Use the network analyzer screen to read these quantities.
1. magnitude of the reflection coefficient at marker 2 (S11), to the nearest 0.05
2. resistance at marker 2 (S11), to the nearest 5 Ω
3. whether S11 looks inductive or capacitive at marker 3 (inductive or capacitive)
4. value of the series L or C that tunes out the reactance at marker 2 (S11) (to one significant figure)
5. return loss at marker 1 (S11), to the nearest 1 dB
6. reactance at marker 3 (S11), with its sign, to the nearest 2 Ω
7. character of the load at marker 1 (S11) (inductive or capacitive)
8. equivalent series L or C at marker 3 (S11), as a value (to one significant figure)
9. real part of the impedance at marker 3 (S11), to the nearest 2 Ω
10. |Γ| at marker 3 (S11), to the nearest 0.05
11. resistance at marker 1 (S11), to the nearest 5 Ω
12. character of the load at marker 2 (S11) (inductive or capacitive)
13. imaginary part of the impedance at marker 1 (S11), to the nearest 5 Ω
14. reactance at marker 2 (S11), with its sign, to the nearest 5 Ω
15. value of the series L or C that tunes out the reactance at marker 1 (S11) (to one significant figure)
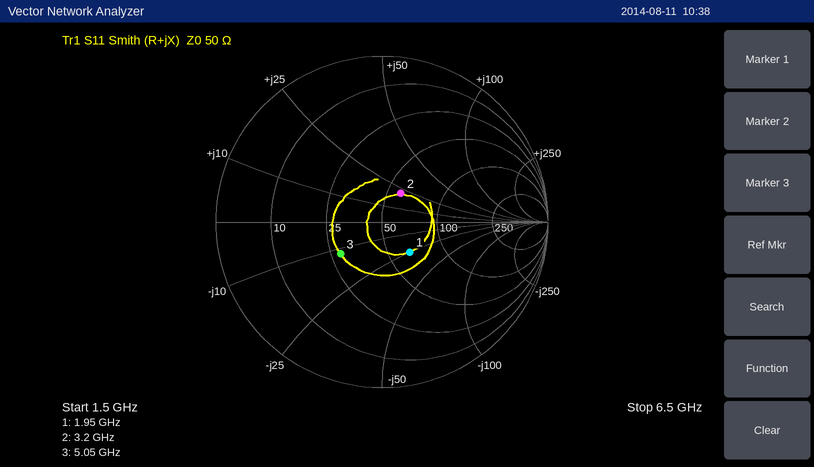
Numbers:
0.20
60 Ω
capacitive
2 pF
12 dB
-12 Ω
capacitive
3 pF
28 Ω
0.30
65 Ω
inductive
-25 Ω
+20 Ω
2 nH
